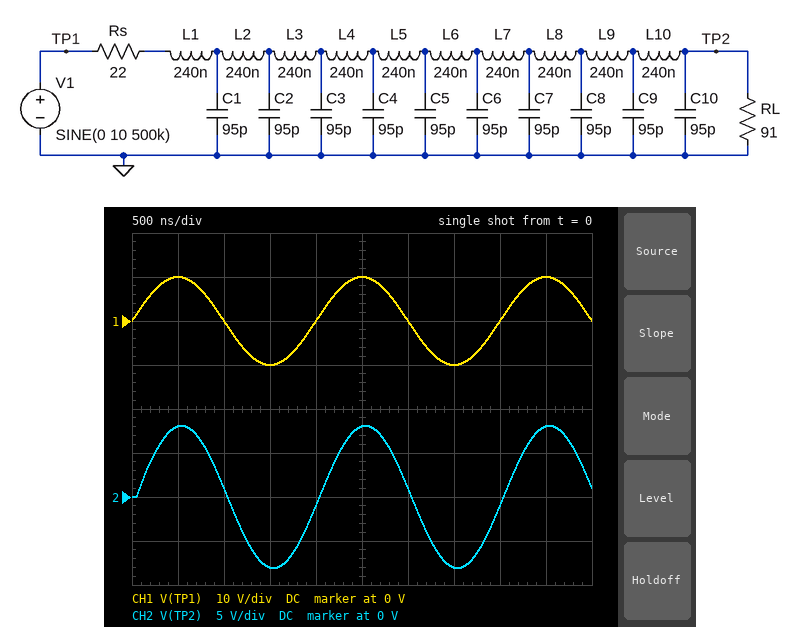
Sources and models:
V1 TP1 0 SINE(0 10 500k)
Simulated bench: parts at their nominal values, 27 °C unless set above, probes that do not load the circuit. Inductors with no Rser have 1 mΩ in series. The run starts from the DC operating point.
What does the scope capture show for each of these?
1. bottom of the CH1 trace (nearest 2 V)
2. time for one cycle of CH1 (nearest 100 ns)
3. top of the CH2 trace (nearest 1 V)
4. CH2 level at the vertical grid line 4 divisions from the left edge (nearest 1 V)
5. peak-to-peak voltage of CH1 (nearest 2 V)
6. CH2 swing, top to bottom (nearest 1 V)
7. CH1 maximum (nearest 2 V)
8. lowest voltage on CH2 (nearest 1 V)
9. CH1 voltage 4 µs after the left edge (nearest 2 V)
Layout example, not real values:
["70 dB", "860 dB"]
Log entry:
["-10 V", "2.0 µs", "8 V", "-1 V", "20 V", "16 V", "10 V", "-8 V", "0 V"]
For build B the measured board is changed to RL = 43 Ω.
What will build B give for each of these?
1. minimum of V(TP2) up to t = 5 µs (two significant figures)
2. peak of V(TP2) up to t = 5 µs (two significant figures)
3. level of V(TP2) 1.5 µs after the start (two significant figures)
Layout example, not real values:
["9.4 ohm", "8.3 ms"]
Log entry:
["-6.6 V", "6.6 V", "-6.5 V"]
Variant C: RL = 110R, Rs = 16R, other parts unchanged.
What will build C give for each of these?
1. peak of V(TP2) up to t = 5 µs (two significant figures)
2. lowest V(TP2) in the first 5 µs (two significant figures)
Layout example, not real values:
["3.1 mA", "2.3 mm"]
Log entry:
["8.8 V", "-8.8 V"]
